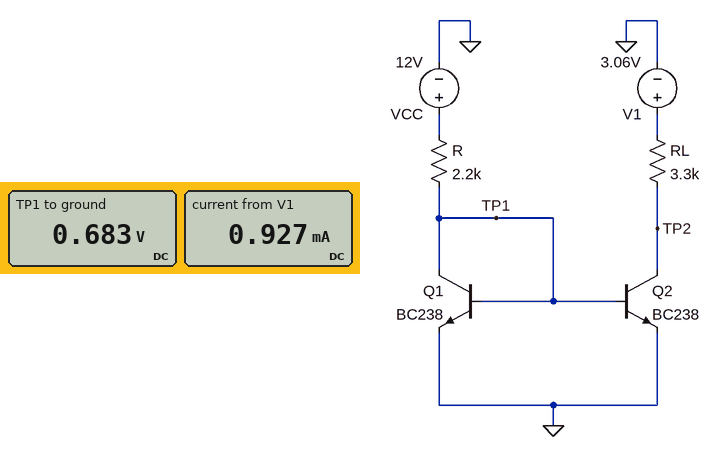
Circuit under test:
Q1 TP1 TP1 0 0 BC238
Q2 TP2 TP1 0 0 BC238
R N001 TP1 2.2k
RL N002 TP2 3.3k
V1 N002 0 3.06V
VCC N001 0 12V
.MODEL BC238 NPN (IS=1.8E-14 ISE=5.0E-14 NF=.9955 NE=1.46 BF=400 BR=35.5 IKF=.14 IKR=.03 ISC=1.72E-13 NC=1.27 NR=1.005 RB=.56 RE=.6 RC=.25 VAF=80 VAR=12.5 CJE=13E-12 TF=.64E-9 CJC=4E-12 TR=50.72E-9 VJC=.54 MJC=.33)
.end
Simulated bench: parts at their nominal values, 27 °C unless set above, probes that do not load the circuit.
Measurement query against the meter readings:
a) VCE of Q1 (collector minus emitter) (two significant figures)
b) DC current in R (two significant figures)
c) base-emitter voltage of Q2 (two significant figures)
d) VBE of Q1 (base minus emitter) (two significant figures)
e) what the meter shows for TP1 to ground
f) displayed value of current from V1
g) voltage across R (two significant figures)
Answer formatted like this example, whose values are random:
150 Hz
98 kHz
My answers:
680 mV
5.1 mA
680 mV
680 mV
0.683 V
0.927 mA
11 V
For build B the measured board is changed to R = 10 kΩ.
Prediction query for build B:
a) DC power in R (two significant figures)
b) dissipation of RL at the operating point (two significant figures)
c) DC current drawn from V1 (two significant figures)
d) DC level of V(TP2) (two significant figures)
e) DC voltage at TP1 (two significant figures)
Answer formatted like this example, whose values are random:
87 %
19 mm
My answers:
13 mW
2.8 mW
910 µA
44 mV
640 mV
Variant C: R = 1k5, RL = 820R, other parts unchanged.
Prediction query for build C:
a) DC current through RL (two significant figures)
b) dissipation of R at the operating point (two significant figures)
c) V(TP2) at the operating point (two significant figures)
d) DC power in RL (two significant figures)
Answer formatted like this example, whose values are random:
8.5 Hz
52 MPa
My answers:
3.7 mA
85 mW
19 mV
11 mW
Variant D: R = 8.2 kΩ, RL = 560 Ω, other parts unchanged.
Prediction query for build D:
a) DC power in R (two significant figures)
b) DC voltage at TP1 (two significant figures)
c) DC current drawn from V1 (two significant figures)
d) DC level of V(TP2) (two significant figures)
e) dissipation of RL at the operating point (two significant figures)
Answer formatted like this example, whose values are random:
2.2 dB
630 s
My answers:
16 mW
650 mV
1.4 mA
2.3 V
1.1 mW
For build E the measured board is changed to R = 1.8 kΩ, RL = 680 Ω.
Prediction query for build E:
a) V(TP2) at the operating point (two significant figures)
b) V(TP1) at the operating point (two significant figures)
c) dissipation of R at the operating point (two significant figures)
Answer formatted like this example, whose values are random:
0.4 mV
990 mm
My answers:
35 mV
690 mV
71 mW
